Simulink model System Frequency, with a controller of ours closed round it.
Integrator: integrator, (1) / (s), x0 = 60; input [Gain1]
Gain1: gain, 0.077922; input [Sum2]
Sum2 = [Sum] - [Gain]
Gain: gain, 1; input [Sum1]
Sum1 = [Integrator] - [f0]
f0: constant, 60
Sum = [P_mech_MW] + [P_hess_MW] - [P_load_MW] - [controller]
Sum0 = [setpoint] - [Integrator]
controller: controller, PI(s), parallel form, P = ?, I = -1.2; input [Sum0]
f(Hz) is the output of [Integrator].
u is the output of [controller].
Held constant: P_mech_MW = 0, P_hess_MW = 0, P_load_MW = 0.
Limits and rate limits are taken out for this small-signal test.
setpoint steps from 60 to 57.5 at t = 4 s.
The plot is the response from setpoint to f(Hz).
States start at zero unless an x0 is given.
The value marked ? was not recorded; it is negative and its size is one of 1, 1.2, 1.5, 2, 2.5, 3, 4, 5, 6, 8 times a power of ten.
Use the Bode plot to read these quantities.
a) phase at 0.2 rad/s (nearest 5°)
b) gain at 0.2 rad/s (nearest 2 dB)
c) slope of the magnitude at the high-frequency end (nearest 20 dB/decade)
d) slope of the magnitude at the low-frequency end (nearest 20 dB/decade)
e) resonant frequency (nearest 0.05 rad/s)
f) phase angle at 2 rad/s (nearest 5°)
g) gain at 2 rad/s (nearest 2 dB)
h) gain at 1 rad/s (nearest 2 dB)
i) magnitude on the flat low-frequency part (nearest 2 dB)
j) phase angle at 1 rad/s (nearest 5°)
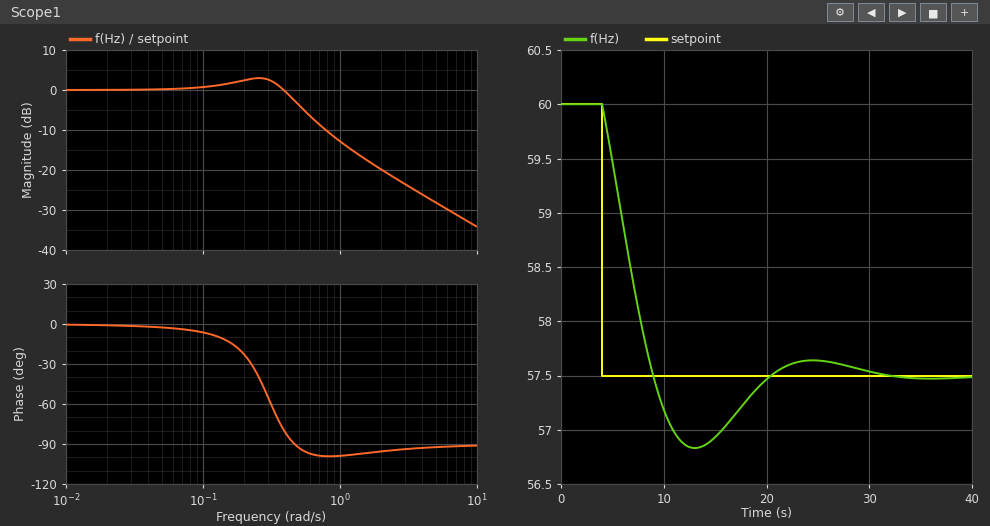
-25°
2 dB
-20 dB/decade
0 dB/decade
0.25 rad/s
-95°
-20 dB
-12 dB
0 dB
-100°
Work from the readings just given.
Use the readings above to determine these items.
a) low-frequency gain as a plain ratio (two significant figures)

1.0
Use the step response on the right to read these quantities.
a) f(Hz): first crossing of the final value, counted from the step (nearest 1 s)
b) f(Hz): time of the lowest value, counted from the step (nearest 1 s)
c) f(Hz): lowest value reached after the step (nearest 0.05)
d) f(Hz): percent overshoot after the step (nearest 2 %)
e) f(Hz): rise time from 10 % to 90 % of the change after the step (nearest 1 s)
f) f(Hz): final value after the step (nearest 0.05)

5 s
9 s
56.85
26 %
4 s
57.50
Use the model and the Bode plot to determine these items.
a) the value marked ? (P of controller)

-2.5
